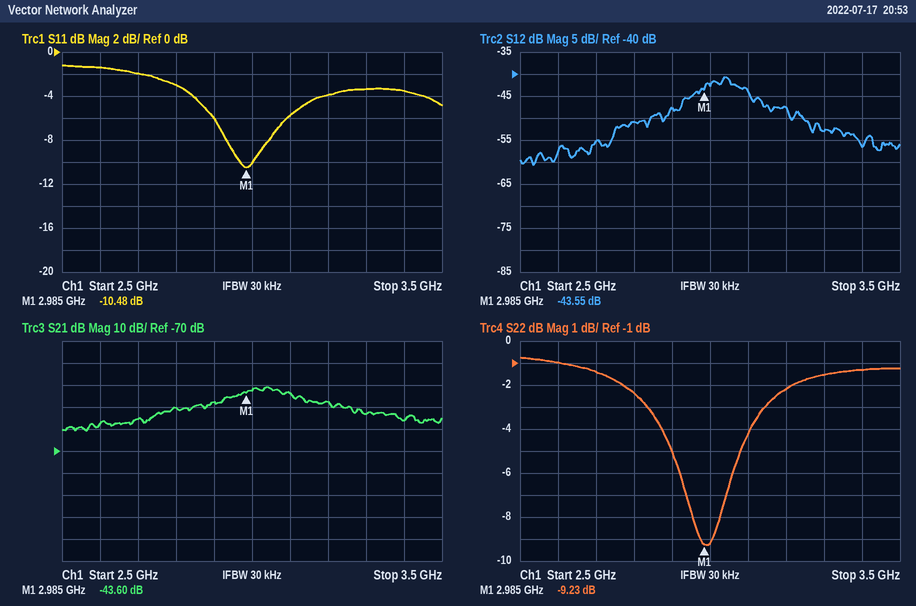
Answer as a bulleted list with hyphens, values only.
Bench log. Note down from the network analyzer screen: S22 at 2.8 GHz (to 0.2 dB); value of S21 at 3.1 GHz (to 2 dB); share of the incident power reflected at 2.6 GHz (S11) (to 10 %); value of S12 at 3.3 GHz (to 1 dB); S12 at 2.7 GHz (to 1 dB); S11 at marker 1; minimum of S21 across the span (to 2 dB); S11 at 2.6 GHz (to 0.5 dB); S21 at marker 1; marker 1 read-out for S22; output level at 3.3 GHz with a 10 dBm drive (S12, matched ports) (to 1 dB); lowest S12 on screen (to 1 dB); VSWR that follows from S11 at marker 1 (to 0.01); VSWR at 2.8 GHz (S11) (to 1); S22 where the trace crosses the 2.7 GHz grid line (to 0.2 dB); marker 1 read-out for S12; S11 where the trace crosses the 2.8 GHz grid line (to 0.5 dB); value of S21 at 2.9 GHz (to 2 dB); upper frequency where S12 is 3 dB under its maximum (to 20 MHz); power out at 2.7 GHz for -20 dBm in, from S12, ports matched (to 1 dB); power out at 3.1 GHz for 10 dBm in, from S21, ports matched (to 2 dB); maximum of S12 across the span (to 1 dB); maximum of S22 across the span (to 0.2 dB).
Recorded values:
- -2.4 dB
- -44 dB
- 70 %
- -53 dB
- -55 dB
- -10.48 dB
- -60 dB
- -1.5 dB
- -43.60 dB
- -9.23 dB
- -43 dBm
- -61 dB
- 1.85
- 6
- -1.4 dB
- -43.55 dB
- -3.0 dB
- -48 dB
- 3.10 GHz
- -75 dBm
- -34 dBm
- -41 dB
- -0.8 dB
